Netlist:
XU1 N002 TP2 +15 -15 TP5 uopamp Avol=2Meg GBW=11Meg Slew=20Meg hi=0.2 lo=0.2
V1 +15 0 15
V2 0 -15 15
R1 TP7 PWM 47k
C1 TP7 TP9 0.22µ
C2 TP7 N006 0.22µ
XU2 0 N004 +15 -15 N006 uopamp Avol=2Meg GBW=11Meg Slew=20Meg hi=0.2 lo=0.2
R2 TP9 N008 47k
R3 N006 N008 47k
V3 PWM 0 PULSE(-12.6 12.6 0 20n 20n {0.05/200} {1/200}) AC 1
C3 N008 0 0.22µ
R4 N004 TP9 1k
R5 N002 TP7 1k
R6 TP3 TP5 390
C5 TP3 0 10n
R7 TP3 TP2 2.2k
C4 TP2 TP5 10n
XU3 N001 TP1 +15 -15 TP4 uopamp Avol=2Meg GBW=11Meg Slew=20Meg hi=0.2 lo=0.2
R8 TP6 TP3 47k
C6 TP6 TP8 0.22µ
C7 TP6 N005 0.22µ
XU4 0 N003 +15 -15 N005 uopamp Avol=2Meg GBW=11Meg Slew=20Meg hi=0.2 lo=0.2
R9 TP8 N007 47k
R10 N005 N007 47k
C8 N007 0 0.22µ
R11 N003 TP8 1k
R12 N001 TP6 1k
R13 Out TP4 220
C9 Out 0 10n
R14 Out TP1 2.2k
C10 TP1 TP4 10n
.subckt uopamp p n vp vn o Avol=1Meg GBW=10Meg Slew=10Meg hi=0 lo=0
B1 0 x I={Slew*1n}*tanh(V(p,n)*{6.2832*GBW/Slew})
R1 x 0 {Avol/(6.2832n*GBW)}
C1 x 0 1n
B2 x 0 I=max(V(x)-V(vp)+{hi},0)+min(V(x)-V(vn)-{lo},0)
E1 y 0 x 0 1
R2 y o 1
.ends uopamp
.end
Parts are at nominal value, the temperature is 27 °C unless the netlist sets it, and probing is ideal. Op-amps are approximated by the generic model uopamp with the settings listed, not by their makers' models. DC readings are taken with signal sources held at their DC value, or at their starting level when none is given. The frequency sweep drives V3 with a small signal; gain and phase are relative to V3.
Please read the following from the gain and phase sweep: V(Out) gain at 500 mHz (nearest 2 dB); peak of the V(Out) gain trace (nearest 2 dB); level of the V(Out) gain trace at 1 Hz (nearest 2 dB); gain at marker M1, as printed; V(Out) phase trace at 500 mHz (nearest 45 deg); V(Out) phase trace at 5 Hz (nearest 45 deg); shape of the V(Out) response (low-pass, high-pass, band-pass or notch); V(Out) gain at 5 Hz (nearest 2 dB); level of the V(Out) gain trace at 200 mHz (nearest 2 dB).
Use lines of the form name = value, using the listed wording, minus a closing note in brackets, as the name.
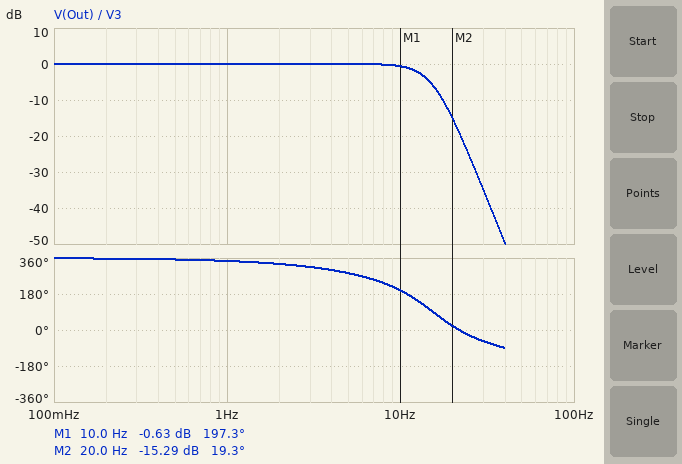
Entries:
V(Out) gain at 500 mHz = 0 dB
peak of the V(Out) gain trace = 0 dB
level of the V(Out) gain trace at 1 Hz = 0 dB
gain at marker M1, as printed = -0.63 dB
V(Out) phase trace at 500 mHz = 360 deg
V(Out) phase trace at 5 Hz = 270 deg
shape of the V(Out) response = low-pass
V(Out) gain at 5 Hz = 0 dB
level of the V(Out) gain trace at 200 mHz = 0 dB
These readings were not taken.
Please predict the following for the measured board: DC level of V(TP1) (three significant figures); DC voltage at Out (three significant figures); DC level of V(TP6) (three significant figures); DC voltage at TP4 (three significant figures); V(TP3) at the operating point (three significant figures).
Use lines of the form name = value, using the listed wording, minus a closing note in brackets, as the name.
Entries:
DC level of V(TP1) = -12.6 V
DC voltage at Out = -12.6 V
DC level of V(TP6) = -12.6 V
DC voltage at TP4 = -12.6 V
V(TP3) at the operating point = -12.6 V
